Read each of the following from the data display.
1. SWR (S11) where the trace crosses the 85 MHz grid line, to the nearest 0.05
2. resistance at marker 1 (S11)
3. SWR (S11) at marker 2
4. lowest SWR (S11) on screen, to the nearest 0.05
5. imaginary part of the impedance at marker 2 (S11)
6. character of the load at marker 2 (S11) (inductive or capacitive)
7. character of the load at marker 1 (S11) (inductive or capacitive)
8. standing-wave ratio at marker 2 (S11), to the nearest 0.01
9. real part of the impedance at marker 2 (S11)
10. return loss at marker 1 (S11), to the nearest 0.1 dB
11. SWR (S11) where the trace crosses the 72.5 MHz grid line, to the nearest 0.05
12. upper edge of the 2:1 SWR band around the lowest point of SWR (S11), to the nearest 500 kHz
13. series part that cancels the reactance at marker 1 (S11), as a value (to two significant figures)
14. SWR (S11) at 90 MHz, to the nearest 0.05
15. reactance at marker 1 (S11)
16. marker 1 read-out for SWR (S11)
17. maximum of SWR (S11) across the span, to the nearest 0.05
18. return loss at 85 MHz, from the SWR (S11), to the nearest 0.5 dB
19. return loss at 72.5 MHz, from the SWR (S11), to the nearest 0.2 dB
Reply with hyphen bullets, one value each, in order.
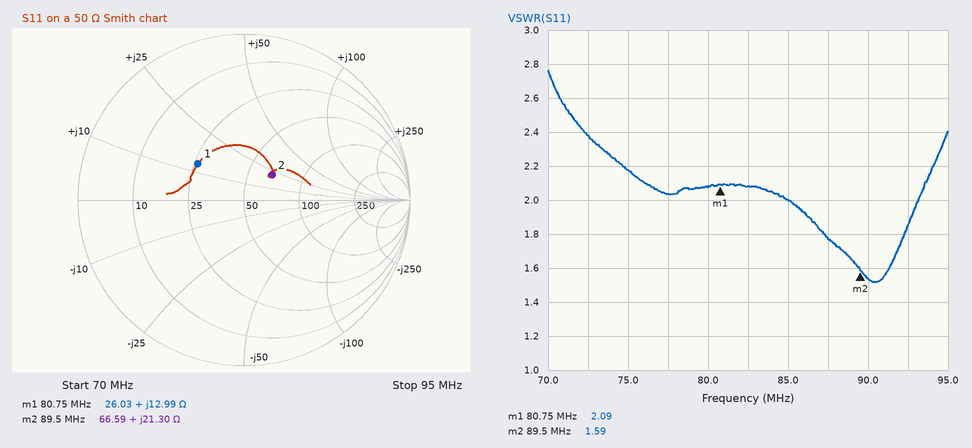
- 2.00
- 26.03 Ω
- 1.59
- 1.50
- +21.30 Ω
- inductive
- inductive
- 1.59
- 66.59 Ω
- 9.0 dB
- 2.40
- 93.0 MHz
- 150 pF
- 1.55
- +12.99 Ω
- 2.09
- 2.75
- 9.5 dB
- 7.8 dB
